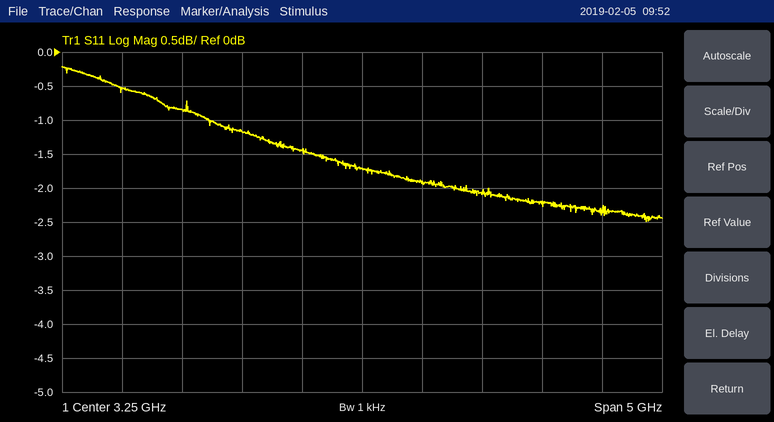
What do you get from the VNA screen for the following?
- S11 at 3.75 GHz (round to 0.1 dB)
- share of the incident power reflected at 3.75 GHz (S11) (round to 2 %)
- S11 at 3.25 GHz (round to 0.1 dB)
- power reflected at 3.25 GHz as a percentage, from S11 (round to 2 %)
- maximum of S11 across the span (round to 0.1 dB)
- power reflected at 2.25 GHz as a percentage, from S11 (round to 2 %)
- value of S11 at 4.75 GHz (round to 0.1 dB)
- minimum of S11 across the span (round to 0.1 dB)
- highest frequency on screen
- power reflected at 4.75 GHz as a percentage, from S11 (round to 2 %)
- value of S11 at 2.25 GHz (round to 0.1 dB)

-1.9 dB
64 %
-1.7 dB
68 %
-0.2 dB
76 %
-2.2 dB
-2.5 dB
5.75 GHz
60 %
-1.2 dB
